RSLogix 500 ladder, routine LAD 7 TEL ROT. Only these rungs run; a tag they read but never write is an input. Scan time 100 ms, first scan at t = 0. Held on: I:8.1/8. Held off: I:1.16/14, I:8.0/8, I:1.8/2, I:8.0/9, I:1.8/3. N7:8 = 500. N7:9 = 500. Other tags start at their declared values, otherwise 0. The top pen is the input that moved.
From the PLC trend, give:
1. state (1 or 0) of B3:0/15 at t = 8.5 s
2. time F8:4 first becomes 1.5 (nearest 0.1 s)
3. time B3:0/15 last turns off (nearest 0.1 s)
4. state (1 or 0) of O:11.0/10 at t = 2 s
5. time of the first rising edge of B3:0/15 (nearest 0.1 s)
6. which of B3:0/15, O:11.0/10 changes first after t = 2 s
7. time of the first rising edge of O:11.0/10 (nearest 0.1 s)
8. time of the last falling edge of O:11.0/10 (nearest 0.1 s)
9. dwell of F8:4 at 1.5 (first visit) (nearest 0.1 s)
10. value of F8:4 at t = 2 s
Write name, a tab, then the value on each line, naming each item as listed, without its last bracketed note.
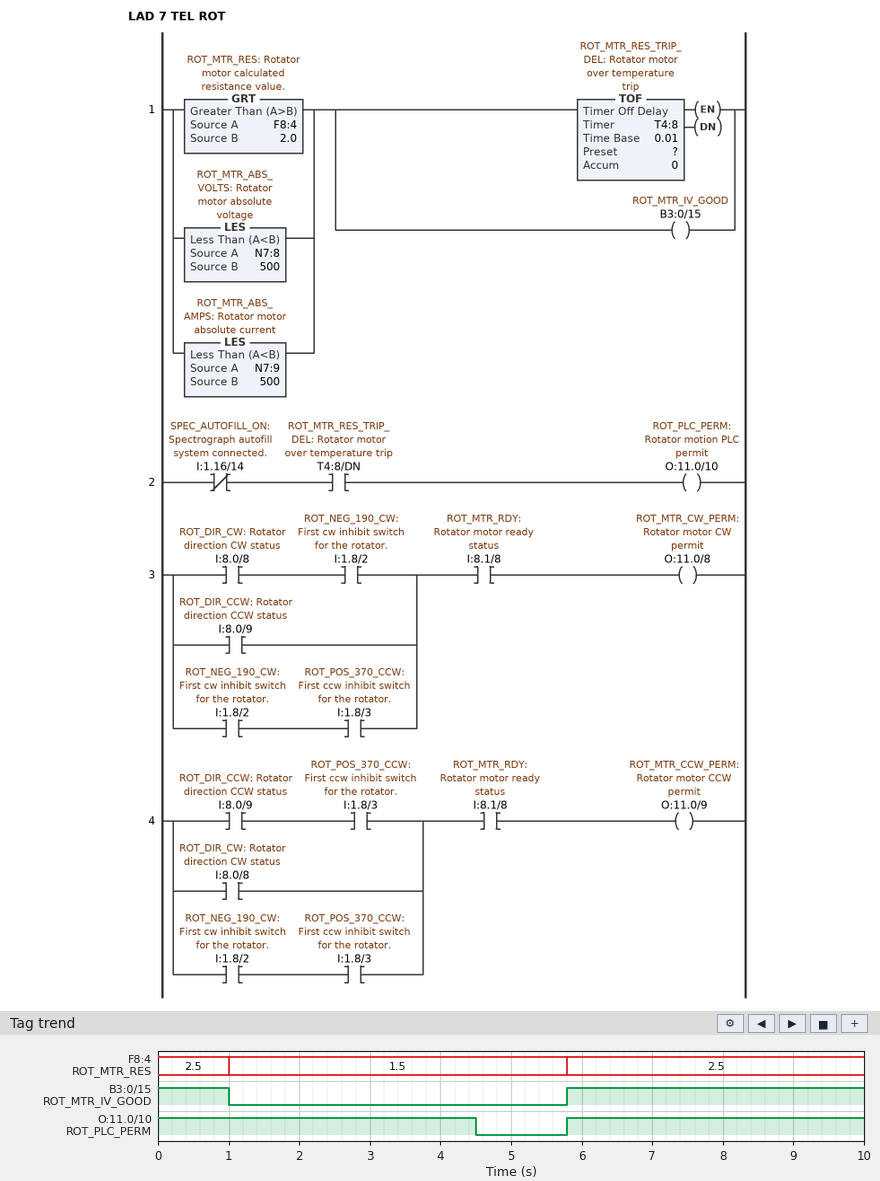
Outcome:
state (1 or 0) of B3:0/15 at t = 8.5 s	1
time F8:4 first becomes 1.5	1.0 s
time B3:0/15 last turns off	1.0 s
state (1 or 0) of O:11.0/10 at t = 2 s	1
time of the first rising edge of B3:0/15	5.8 s
which of B3:0/15, O:11.0/10 changes first after t = 2 s	O:11.0/10
time of the first rising edge of O:11.0/10	5.8 s
time of the last falling edge of O:11.0/10	4.5 s
dwell of F8:4 at 1.5 (first visit)	4.8 s
value of F8:4 at t = 2 s	1.5
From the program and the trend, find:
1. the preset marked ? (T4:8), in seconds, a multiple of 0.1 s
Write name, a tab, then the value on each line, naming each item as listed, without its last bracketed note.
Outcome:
the preset marked ? (T4:8), in seconds, a multiple of 0.1 s	3.5 s
